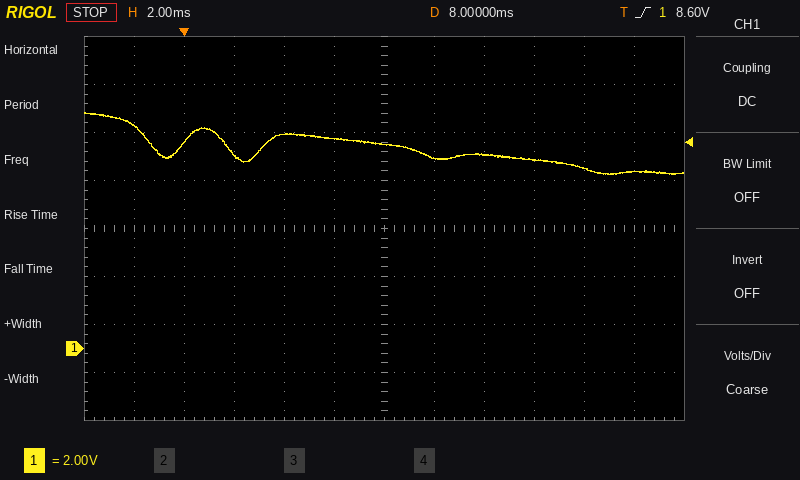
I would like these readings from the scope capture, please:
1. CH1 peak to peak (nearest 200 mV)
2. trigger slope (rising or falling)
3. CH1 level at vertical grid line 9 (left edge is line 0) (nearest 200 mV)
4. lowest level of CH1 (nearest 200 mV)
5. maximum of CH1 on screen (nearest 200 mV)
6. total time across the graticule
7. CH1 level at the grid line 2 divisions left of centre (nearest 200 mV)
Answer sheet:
2.6 V
rising
7.8 V
7.2 V
9.8 V
24 ms
9.0 V
